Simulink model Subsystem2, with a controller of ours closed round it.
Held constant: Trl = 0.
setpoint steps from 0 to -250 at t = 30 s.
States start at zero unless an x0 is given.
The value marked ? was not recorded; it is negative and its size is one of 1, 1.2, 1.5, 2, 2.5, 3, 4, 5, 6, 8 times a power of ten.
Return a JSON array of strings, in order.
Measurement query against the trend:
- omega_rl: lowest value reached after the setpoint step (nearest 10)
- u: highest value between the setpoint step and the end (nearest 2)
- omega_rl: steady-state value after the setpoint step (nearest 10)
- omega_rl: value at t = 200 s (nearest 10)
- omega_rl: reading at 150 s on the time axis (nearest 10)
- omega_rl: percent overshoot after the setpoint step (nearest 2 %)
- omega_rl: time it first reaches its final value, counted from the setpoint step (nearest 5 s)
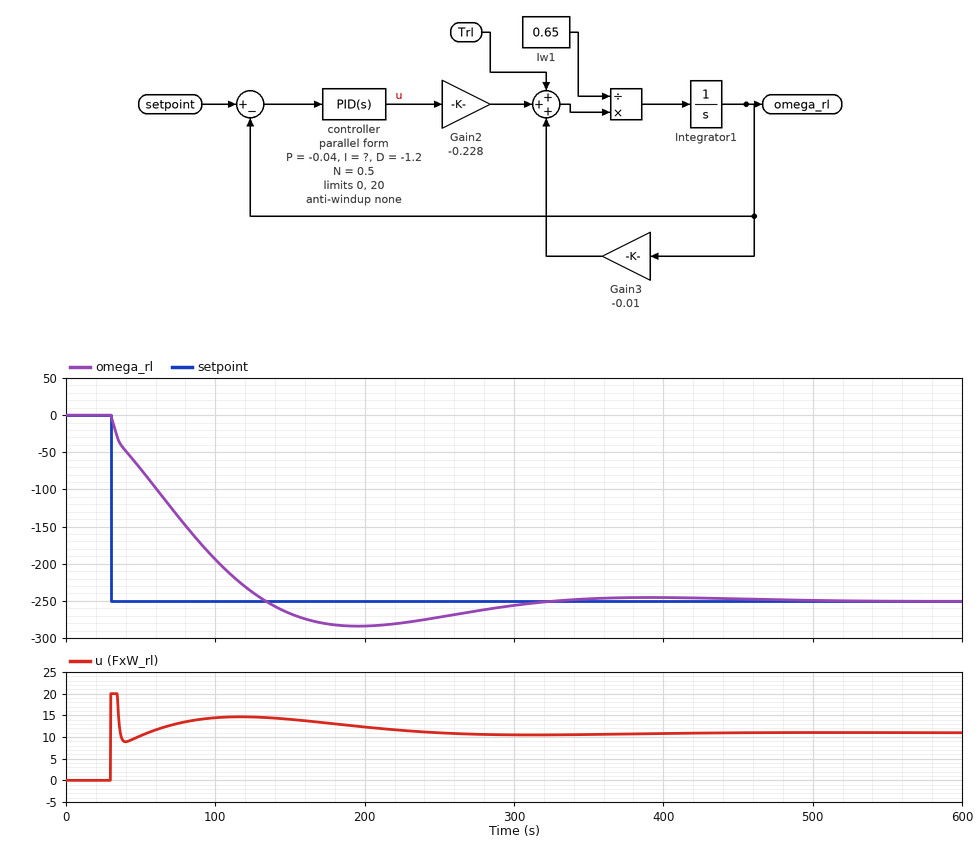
["-280", "20", "-250", "-280", "-270", "14 %", "105 s"]
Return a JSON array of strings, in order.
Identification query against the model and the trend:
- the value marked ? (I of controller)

["-0.0015"]
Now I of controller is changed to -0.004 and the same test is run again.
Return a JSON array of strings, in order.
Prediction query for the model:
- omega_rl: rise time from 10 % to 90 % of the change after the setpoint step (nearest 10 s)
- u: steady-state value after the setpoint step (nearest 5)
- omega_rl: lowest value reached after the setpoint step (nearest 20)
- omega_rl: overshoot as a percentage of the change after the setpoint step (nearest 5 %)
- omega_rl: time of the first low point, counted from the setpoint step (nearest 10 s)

["50 s", "10", "-320", "30 %", "100 s"]
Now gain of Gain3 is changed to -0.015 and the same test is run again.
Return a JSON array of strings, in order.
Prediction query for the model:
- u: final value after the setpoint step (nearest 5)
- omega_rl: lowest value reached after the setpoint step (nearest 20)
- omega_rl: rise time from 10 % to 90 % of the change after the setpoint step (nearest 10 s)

["15", "-260", "100 s"]
